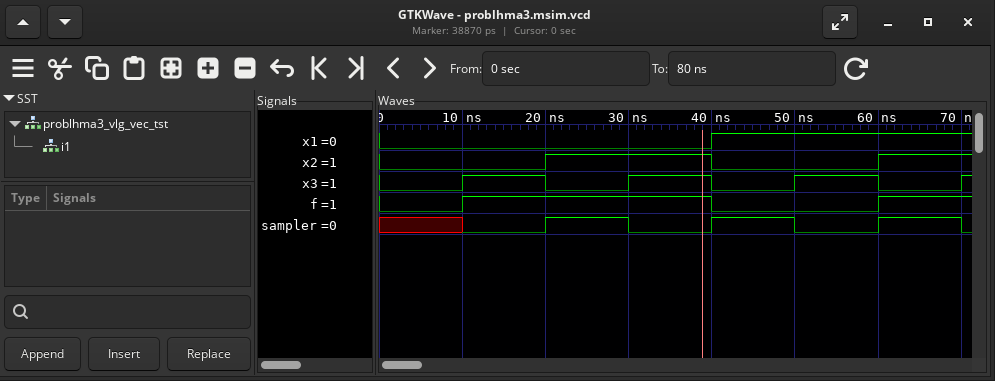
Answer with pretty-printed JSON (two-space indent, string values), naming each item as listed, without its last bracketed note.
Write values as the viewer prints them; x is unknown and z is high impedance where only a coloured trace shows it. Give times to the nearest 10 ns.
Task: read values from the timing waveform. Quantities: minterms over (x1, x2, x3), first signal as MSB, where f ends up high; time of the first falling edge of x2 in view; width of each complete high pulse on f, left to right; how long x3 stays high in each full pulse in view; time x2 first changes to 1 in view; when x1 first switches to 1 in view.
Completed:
{
  "minterms over (x1, x2, x3), first signal as MSB, where f ends up high": "1, 2, 3, 6, 7",
  "time of the first falling edge of x2 in view": "40 ns",
  "width of each complete high pulse on f, left to right": "30 ns",
  "how long x3 stays high in each full pulse in view": "10 ns, 10 ns, 10 ns",
  "time x2 first changes to 1 in view": "20 ns",
  "when x1 first switches to 1 in view": "40 ns"
}
